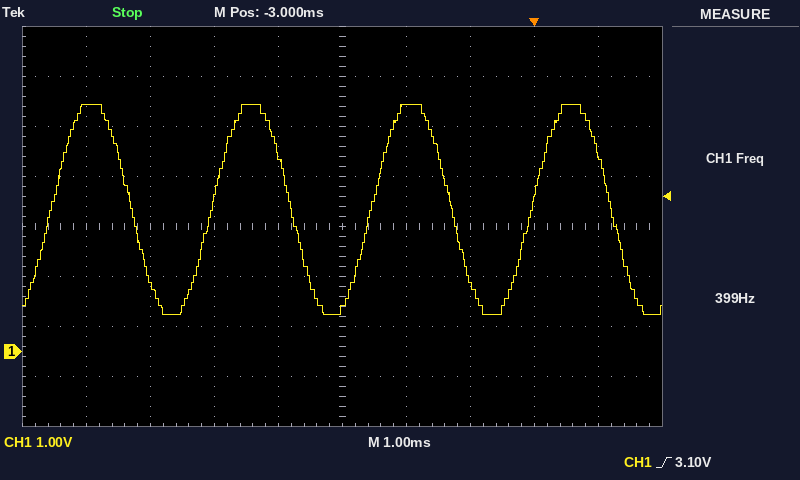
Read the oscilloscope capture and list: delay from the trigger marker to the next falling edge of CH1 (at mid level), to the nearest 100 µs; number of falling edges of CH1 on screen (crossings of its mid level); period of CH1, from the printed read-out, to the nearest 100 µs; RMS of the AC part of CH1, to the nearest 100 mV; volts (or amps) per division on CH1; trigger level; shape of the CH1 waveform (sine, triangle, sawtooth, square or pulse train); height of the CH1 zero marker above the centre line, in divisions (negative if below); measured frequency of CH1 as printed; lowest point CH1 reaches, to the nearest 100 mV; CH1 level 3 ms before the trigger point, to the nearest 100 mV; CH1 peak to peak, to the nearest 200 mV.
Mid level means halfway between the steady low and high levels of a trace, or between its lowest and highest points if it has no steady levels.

1.2 ms
4
2.5 ms
1.5 V
1 V
3.10 V
sine
-2.5 div
399 Hz
700 mV
800 mV
4.2 V
